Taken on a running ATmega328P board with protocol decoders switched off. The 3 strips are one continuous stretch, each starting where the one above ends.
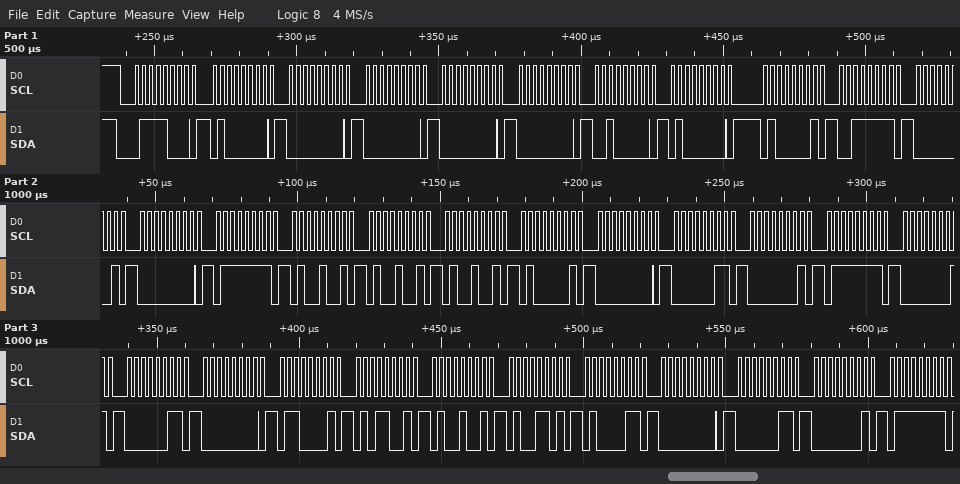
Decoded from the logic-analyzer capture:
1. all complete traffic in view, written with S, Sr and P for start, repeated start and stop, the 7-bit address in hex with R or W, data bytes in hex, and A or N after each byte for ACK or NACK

S 3CW A 40 A 00 A 00 A 00 A 00 A 20 A 40 A 41 A 3F A 01 A 00 A 7F A 49 A 49 A 49 A 41 A 00 A 03 A 01 A 7F A 01 A 03 A 00 A 61 A 59 A 49 A 4D A 43 A 00 A 03 A 01 A 7F A
